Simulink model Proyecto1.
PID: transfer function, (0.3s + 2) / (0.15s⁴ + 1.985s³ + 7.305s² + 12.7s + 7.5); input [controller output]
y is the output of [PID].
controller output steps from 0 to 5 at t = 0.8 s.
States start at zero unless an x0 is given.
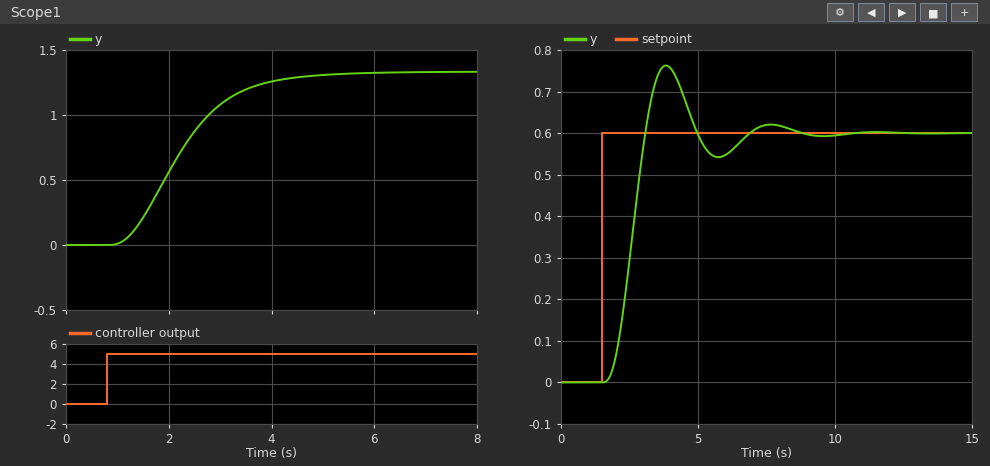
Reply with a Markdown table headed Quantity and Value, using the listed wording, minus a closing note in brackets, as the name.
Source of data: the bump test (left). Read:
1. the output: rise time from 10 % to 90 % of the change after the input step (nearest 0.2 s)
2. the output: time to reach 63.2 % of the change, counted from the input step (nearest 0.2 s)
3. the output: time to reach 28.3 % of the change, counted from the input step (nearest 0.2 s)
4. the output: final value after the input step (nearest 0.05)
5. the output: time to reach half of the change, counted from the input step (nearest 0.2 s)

| Quantity | Value |
|---|---|
| the output: rise time from 10 % to 90 % of the change after the input step | 2.2 s |
| the output: time to reach 63.2 % of the change, counted from the input step | 1.6 s |
| the output: time to reach 28.3 % of the change, counted from the input step | 1.0 s |
| the output: final value after the input step | 1.35 |
| the output: time to reach half of the change, counted from the input step | 1.4 s |
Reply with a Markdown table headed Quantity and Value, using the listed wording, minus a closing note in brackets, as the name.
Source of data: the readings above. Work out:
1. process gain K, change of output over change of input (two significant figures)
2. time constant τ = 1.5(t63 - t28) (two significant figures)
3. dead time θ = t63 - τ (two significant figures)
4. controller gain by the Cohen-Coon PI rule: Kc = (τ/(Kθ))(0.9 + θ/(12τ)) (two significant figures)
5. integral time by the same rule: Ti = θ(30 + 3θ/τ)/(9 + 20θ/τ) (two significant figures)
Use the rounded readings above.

| Quantity | Value |
|---|---|
| process gain K, change of output over change of input | 0.27 |
| time constant τ = 1.5(t63 - t28) | 0.90 s |
| dead time θ = t63 - τ | 0.70 s |
| controller gain by the Cohen-Coon PI rule: Kc = (τ/(Kθ))(0.9 + θ/(12τ)) | 4.6 |
| integral time by the same rule: Ti = θ(30 + 3θ/τ)/(9 + 20θ/τ) | 0.92 s |
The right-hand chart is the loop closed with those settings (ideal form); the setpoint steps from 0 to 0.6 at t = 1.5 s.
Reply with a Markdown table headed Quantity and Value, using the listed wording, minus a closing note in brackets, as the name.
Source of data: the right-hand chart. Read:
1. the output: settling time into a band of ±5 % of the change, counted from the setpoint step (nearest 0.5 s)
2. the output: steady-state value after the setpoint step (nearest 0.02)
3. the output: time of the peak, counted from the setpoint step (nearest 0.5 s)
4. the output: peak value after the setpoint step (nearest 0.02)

| Quantity | Value |
|---|---|
| the output: settling time into a band of ±5 % of the change, counted from the setpoint step | 5.0 s |
| the output: steady-state value after the setpoint step | 0.60 |
| the output: time of the peak, counted from the setpoint step | 2.5 s |
| the output: peak value after the setpoint step | 0.76 |
